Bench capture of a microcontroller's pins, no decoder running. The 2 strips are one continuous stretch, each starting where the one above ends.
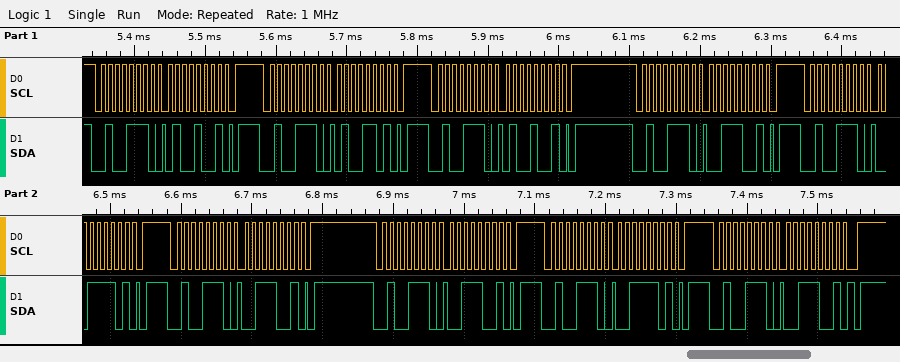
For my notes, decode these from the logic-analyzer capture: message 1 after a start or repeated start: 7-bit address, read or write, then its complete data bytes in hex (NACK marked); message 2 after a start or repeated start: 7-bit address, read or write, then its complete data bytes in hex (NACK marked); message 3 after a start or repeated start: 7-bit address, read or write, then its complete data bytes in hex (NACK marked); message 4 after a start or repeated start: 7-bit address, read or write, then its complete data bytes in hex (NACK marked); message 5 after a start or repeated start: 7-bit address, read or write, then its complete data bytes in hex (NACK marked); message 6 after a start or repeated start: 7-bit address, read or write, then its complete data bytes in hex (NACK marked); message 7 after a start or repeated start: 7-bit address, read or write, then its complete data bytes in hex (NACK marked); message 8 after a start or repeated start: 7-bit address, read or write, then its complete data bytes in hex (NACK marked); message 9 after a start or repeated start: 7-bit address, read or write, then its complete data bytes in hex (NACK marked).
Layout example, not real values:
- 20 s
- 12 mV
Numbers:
- 0x27 write: 49
- 0x27 write: 4D
- 0x27 write: 49
- 0x27 write: 39
- 0x27 write: 3D
- 0x27 write: 39
- 0x27 write: 39
- 0x27 write: 3D
- 0x27 write: 39
